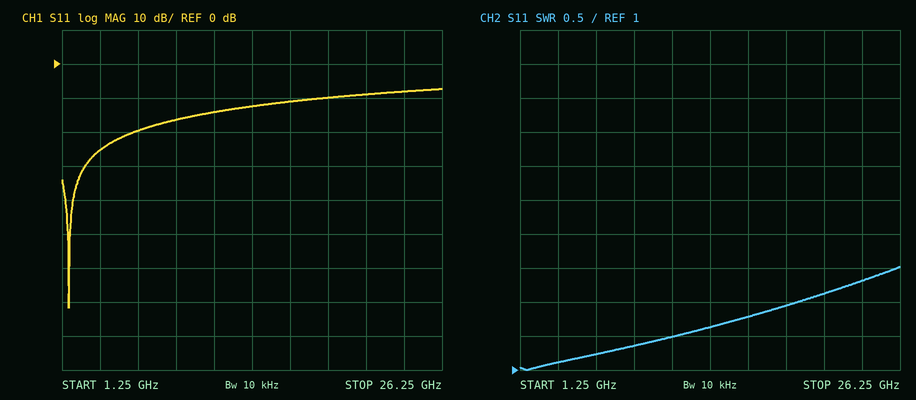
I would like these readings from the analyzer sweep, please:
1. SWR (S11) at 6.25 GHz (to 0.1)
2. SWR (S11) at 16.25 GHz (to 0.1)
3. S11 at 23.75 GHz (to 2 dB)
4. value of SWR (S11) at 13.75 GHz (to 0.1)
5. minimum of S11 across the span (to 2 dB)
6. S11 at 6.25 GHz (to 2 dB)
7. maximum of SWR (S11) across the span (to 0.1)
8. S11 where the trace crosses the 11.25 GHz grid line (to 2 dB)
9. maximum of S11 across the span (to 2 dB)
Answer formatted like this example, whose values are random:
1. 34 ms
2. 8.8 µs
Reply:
1. 1.2
2. 1.8
3. -8 dB
4. 1.6
5. -72 dB
6. -20 dB
7. 2.5
8. -14 dB
9. -8 dB
